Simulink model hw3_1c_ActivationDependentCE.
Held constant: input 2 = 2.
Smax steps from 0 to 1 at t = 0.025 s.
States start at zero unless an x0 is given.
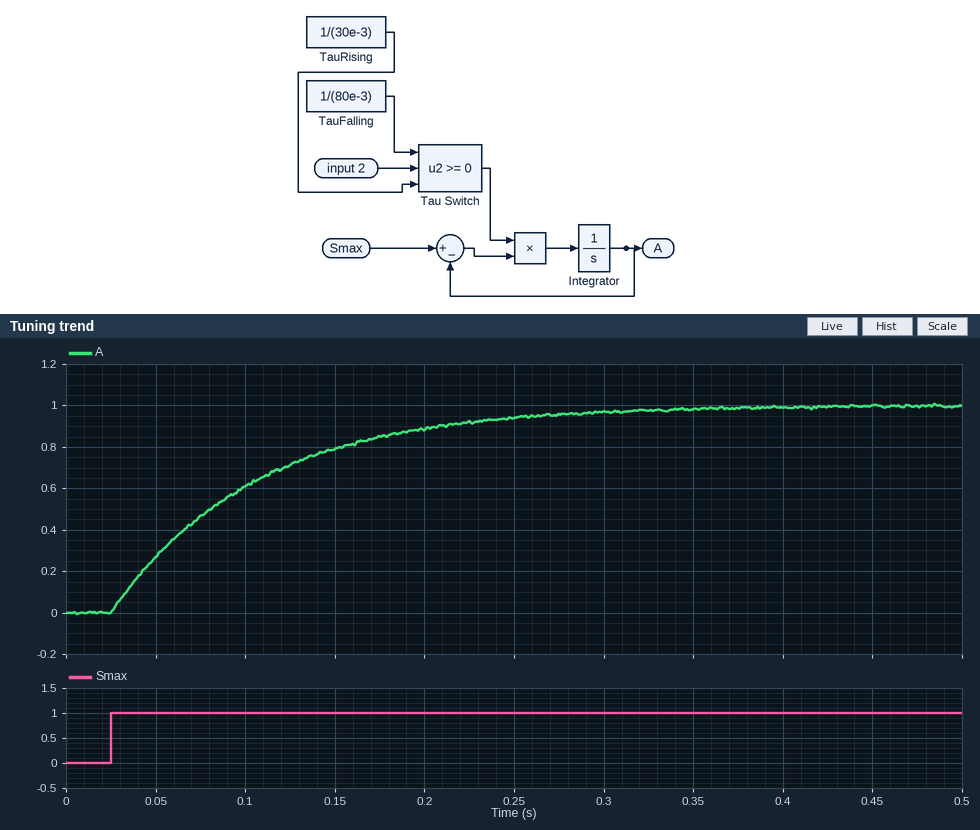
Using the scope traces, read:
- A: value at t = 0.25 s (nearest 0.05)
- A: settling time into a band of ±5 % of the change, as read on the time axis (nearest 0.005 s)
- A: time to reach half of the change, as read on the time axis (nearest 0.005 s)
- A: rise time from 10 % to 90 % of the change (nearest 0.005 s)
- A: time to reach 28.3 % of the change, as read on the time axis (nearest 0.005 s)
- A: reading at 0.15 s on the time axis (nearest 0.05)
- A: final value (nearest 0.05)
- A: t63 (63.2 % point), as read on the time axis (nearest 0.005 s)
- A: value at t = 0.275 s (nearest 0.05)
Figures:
0.95
0.265 s
0.080 s
0.175 s
0.050 s
0.80
1.00
0.105 s
0.95
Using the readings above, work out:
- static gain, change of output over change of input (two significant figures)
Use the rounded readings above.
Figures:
1.0
